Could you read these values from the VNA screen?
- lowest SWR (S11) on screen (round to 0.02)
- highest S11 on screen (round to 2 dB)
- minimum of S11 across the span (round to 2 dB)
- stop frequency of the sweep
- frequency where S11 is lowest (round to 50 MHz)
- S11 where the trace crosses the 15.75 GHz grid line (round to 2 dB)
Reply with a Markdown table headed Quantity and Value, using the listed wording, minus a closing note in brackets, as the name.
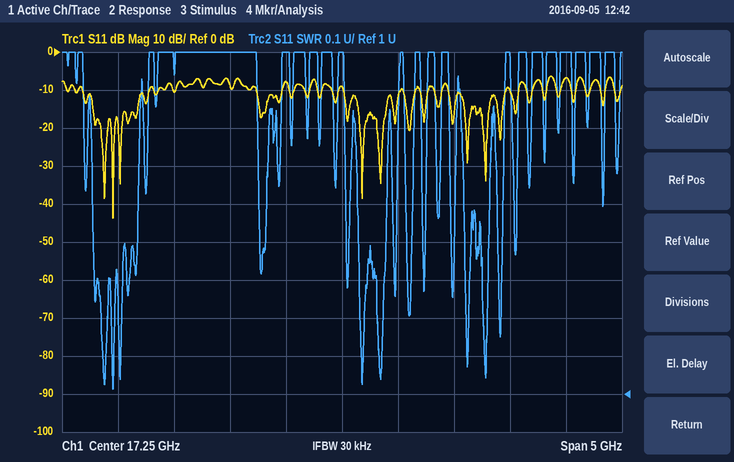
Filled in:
| Quantity | Value |
|---|---|
| lowest SWR (S11) on screen | 1.02 |
| highest S11 on screen | -6 dB |
| minimum of S11 across the span | -44 dB |
| stop frequency of the sweep | 19.75 GHz |
| frequency where S11 is lowest | 15.20 GHz |
| S11 where the trace crosses the 15.75 GHz grid line | -10 dB |
